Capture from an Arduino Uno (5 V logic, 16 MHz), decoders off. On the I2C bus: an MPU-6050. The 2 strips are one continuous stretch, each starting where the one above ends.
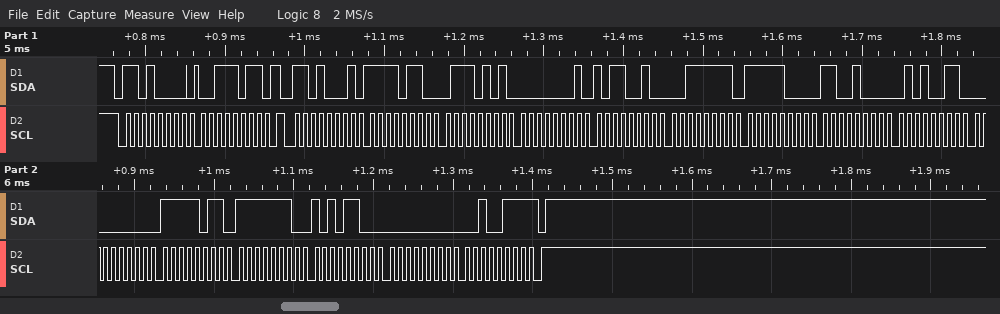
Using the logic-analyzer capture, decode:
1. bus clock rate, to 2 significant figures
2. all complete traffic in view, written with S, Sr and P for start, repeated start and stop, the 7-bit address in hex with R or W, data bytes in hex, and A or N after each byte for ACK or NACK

100 kHz
S 68W A 3B A Sr 68R A F6 A 75 A 01 A B2 A 3F A F8 A C8 A 53 A 00 A FB A FE A AC A 00 A 27 N P
